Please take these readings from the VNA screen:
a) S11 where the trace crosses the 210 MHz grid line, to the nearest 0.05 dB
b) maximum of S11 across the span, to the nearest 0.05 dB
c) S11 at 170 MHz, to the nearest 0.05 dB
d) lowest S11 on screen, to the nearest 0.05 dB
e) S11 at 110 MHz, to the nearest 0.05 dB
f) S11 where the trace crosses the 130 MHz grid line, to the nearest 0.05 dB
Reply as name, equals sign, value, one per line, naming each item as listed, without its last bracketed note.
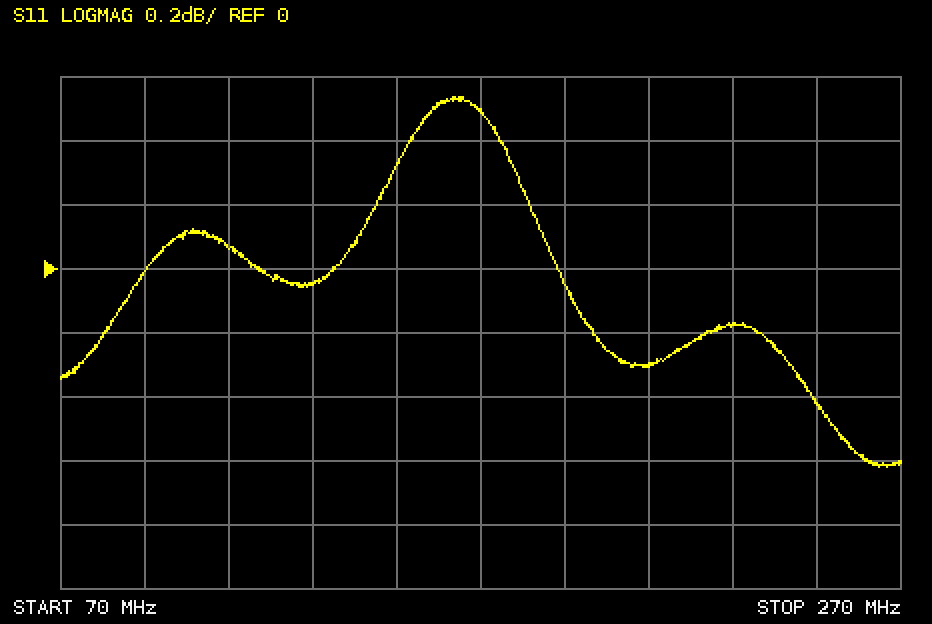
S11 where the trace crosses the 210 MHz grid line, to the nearest 0.05 dB = -0.30 dB
maximum of S11 across the span, to the nearest 0.05 dB = 0.55 dB
S11 at 170 MHz, to the nearest 0.05 dB = 0.50 dB
lowest S11 on screen, to the nearest 0.05 dB = -0.60 dB
S11 at 110 MHz, to the nearest 0.05 dB = 0.05 dB
S11 where the trace crosses the 130 MHz grid line, to the nearest 0.05 dB = -0.05 dB
